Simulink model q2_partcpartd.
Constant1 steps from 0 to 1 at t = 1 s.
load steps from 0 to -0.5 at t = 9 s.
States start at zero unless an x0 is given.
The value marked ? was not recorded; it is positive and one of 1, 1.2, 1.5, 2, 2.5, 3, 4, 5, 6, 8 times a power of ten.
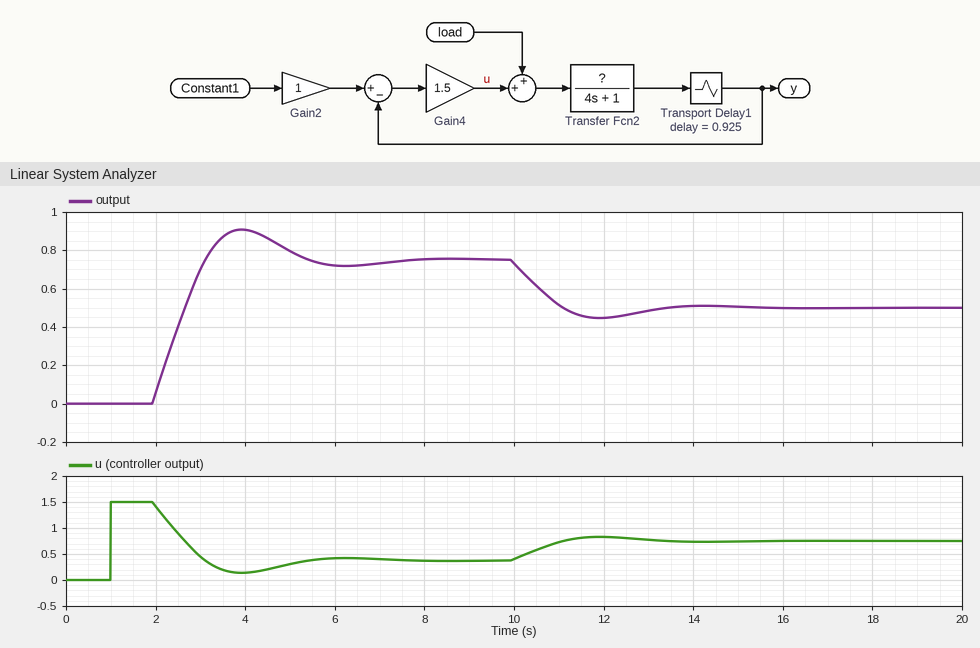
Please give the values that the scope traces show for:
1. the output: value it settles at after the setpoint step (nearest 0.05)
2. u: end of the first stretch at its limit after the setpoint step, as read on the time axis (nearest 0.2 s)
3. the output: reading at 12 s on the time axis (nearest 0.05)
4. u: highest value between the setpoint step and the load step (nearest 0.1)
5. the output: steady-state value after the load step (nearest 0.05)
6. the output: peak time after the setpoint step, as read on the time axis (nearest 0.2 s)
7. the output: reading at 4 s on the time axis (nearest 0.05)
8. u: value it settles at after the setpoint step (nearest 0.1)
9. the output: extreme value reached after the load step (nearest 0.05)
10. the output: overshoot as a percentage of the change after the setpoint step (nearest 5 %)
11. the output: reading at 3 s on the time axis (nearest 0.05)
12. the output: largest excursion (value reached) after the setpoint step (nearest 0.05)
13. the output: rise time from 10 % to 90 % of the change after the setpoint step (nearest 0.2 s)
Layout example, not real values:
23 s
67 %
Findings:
0.75
2.0 s
0.45
1.5
0.50
4.0 s
0.90
0.4
0.45
20 %
0.70
0.90
1.0 s
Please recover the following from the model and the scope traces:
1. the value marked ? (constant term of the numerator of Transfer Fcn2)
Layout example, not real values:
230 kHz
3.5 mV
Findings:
2
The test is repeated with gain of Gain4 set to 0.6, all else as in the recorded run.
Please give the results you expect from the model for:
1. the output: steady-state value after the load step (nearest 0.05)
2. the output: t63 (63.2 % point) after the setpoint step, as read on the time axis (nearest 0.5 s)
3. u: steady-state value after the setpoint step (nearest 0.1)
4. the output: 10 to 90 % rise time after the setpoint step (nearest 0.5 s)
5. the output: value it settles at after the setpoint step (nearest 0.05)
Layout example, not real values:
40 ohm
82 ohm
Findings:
0.10
3.5 s
0.3
2.5 s
0.55
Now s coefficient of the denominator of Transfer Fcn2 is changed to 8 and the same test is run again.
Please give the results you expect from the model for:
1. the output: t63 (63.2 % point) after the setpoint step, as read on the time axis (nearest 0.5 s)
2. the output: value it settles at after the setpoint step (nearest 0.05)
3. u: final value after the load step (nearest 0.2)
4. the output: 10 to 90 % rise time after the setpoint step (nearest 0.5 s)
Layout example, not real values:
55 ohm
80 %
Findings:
3.5 s
0.75
0.8
2.5 s
